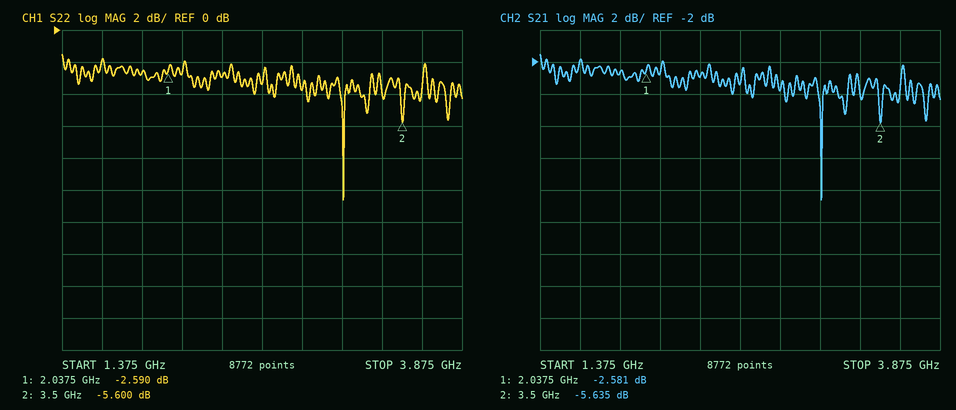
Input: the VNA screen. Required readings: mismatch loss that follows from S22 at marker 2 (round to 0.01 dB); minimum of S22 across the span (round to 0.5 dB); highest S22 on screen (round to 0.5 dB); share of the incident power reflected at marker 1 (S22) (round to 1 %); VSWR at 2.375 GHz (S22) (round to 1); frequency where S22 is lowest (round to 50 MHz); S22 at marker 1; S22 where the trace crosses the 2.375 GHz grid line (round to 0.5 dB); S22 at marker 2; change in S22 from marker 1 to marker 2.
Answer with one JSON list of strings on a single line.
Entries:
["1.40 dB", "-10.5 dB", "-1.5 dB", "55 %", "6", "3.15 GHz", "-2.590 dB", "-3.0 dB", "-5.600 dB", "-3.010 dB"]
